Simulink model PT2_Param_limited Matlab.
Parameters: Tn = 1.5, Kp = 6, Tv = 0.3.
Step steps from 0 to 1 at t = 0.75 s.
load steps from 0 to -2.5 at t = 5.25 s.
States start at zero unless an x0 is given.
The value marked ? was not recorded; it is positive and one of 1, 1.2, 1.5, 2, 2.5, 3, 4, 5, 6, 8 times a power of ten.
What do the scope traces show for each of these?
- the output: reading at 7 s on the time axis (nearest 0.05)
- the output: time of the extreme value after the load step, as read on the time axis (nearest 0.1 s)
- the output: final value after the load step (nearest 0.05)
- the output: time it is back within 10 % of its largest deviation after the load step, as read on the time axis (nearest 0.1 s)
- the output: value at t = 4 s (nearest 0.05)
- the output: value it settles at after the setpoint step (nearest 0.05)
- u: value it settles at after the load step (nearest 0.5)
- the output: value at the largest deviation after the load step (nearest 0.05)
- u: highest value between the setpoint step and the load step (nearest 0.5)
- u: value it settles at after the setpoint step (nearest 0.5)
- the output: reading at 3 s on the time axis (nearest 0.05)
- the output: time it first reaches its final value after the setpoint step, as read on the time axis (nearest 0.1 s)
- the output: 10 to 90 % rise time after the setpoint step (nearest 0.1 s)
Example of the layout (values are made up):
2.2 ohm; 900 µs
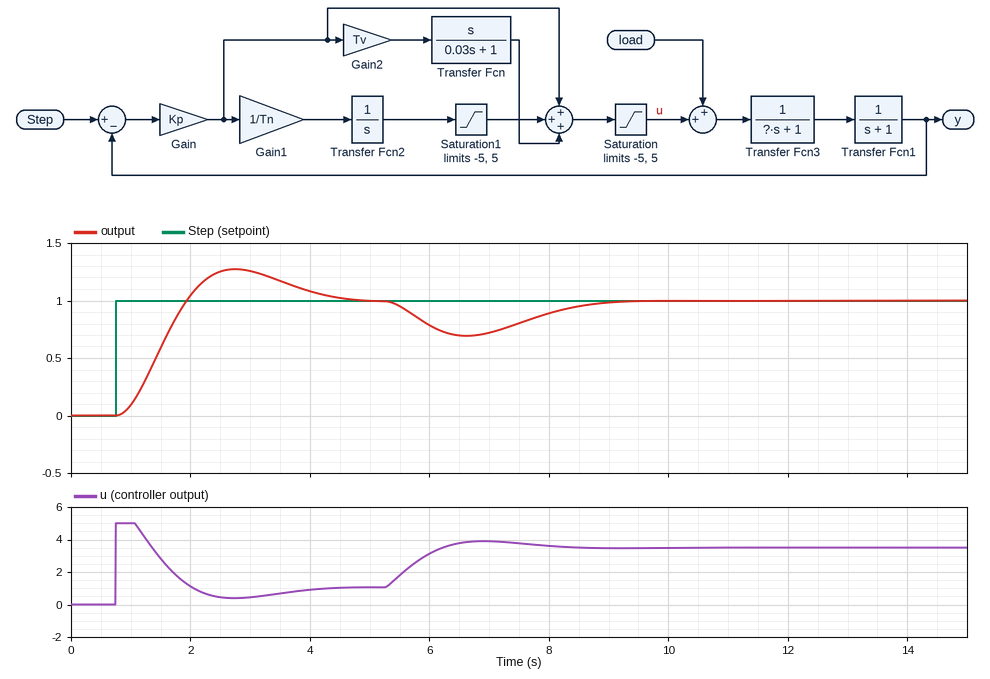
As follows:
0.70; 6.6 s; 1.00; 8.8 s; 1.10; 1.00; 3.5; 0.70; 5.0; 1.0; 1.25; 1.9 s; 0.8 s
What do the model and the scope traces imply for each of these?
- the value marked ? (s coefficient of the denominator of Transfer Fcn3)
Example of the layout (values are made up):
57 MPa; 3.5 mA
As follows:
1.5
